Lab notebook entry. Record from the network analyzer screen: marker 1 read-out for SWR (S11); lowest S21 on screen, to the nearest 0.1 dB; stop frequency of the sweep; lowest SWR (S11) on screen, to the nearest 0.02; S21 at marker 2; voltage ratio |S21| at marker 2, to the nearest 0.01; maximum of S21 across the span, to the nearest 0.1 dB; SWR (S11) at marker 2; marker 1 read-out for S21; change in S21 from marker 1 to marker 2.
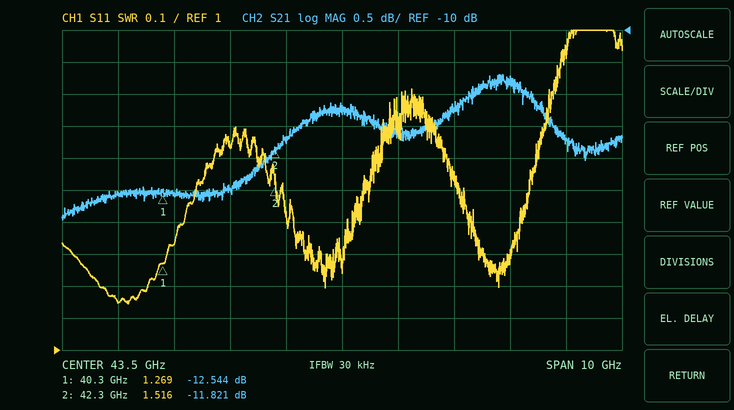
1.269
-13.0 dB
48.5 GHz
1.14
-11.821 dB
0.26
-10.7 dB
1.516
-12.544 dB
0.723 dB
